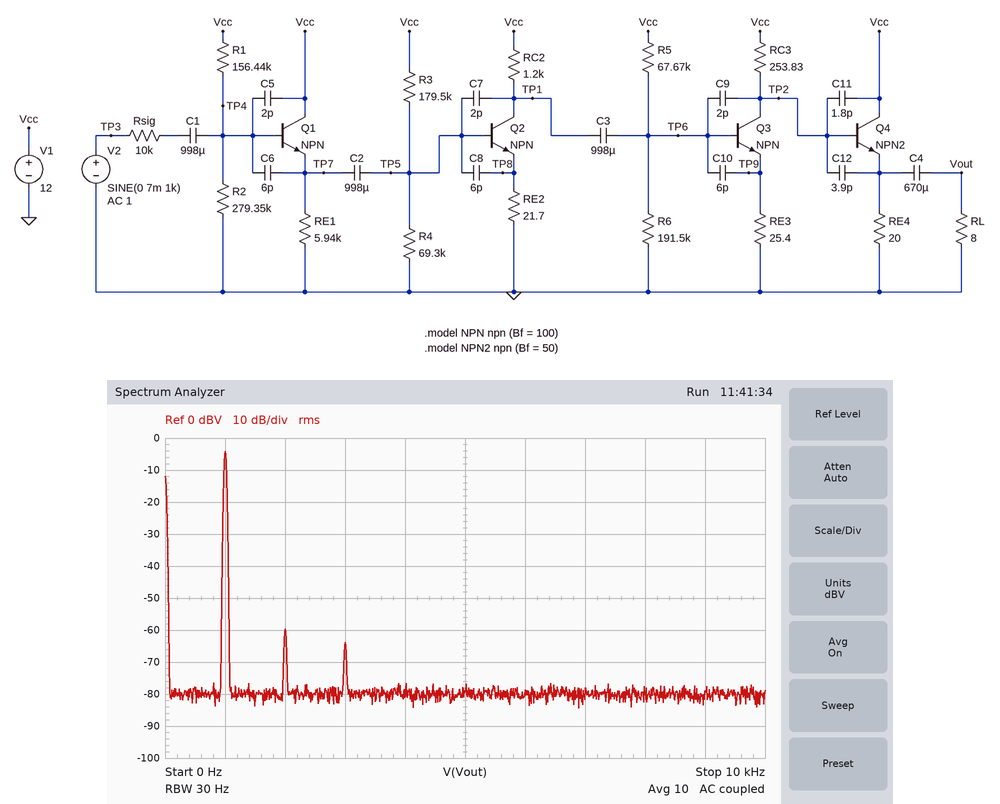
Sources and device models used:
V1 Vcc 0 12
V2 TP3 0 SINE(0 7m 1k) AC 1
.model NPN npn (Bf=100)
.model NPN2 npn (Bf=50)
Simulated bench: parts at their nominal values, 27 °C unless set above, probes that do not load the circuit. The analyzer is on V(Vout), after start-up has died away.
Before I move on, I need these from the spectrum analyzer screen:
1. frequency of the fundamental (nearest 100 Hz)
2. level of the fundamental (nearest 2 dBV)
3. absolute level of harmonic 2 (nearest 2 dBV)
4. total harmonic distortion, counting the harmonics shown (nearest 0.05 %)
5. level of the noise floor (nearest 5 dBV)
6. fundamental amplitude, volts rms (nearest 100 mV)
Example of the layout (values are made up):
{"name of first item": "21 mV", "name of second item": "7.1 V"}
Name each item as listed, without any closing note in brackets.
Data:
{"frequency of the fundamental": "1.0 kHz", "level of the fundamental": "-4 dBV", "absolute level of harmonic 2": "-60 dBV", "total harmonic distortion, counting the harmonics shown": "0.15 %", "level of the noise floor": "-80 dBV", "fundamental amplitude, volts rms": "600 mV"}
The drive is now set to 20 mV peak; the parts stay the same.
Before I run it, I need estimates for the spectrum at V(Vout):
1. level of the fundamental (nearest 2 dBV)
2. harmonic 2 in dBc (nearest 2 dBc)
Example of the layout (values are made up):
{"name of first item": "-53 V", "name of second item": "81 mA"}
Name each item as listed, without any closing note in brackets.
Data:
{"level of the fundamental": "4 dBV", "harmonic 2 in dBc": "-24 dBc"}
